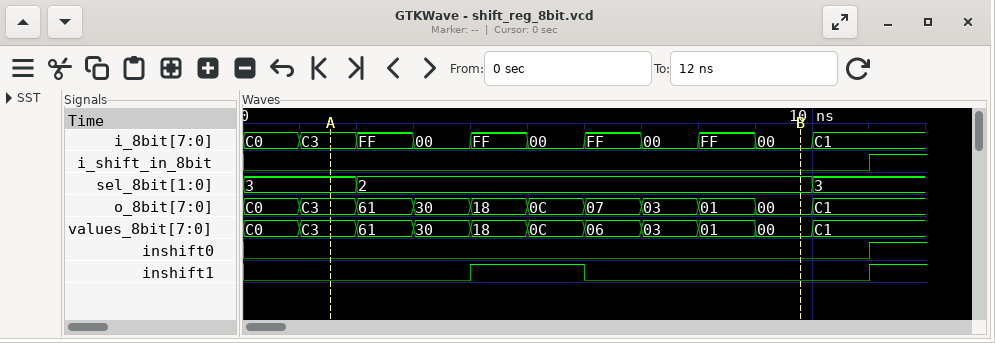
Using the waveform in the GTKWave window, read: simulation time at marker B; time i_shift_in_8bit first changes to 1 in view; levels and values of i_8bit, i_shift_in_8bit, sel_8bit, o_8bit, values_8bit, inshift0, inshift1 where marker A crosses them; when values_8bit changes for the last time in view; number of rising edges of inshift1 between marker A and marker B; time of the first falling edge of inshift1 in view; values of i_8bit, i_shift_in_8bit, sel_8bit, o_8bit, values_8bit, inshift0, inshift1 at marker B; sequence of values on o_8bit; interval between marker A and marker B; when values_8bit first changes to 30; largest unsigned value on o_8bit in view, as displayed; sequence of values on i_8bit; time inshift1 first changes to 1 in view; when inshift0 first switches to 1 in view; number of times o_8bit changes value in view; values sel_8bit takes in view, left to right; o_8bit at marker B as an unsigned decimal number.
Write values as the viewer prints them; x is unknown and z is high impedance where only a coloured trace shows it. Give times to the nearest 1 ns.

10 ns
11 ns
i_8bit=C3, i_shift_in_8bit=0, sel_8bit=3, o_8bit=C3, values_8bit=C3, inshift0=0, inshift1=0
10 ns
1
6 ns
i_8bit=00, i_shift_in_8bit=0, sel_8bit=2, o_8bit=00, values_8bit=00, inshift0=0, inshift1=0
C0, C3, 61, 30, 18, 0C, 07, 03, 01, 00, C1
8 ns
3 ns
C3
C0, C3, FF, 00, FF, 00, FF, 00, FF, 00, C1
4 ns
11 ns
10
3, 2, 3
0
